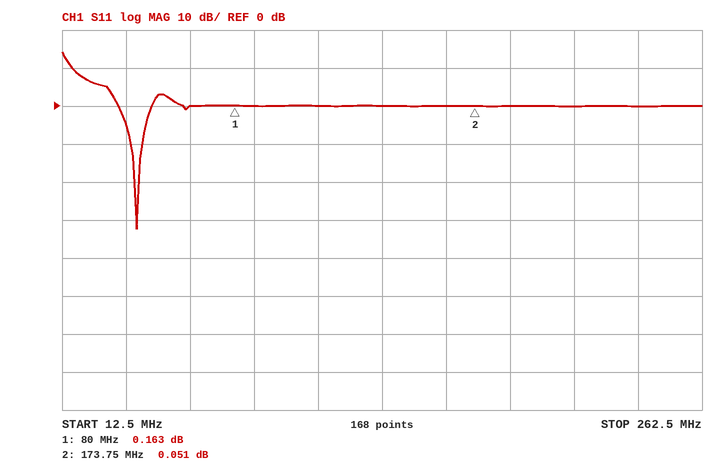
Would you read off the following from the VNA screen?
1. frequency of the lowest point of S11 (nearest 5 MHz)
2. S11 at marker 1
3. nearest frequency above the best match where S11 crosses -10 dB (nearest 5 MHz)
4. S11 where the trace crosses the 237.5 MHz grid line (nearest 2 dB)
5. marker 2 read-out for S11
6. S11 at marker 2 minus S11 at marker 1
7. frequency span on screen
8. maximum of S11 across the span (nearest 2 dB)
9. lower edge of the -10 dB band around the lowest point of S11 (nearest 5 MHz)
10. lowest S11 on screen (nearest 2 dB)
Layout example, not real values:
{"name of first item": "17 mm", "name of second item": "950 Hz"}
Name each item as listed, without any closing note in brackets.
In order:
{"frequency of the lowest point of S11": "40 MHz", "S11 at marker 1": "0.163 dB", "nearest frequency above the best match where S11 crosses -10 dB": "45 MHz", "S11 where the trace crosses the 237.5 MHz grid line": "0 dB", "marker 2 read-out for S11": "0.051 dB", "S11 at marker 2 minus S11 at marker 1": "-0.112 dB", "frequency span on screen": "250 MHz", "maximum of S11 across the span": "14 dB", "lower edge of the -10 dB band around the lowest point of S11": "40 MHz", "lowest S11 on screen": "-32 dB"}
